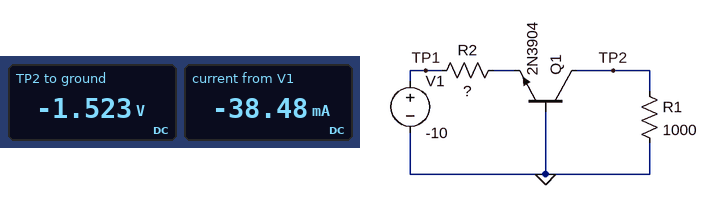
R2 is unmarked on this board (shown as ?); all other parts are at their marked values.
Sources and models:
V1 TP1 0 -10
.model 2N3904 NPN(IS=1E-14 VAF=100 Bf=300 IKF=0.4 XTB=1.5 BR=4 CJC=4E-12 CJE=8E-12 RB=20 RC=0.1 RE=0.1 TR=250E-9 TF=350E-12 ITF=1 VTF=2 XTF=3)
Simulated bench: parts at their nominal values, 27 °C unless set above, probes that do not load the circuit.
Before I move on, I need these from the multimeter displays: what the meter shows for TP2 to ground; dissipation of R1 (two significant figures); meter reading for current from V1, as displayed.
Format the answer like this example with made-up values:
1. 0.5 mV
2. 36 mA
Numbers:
1. -1.523 V
2. 2.3 mW
3. -38.48 mA
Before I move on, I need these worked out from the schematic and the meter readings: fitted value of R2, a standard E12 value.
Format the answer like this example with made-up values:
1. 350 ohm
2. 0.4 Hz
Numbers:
1. 220 Ω
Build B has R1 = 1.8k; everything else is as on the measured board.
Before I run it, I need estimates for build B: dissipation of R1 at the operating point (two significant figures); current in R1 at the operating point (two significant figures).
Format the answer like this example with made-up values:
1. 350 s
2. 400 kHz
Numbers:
1. 1.3 mW
2. 850 µA
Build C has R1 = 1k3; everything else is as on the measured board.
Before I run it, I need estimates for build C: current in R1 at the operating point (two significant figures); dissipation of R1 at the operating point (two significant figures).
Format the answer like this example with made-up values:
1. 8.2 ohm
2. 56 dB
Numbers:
1. 1.2 mA
2. 1.8 mW
